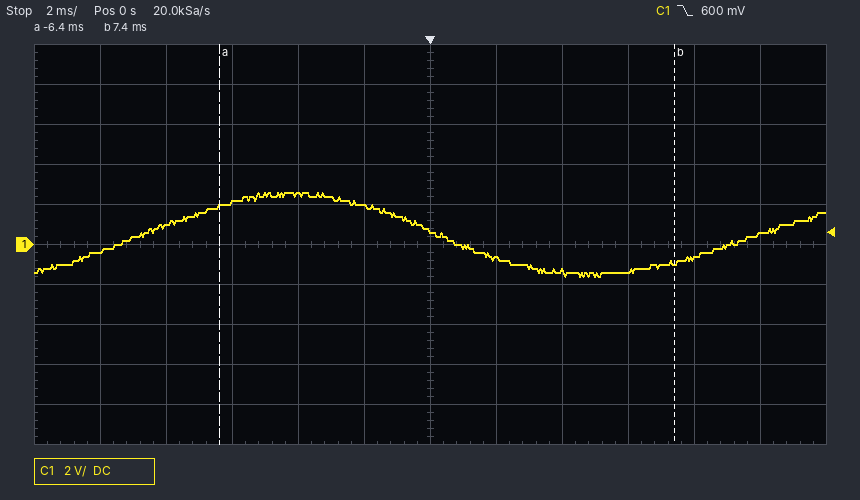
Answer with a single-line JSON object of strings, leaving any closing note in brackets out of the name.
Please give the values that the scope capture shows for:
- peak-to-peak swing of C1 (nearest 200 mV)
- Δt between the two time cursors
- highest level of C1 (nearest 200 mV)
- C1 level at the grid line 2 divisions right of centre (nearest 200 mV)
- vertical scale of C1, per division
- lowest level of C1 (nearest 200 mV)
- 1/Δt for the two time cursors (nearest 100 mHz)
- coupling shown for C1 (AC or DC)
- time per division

{"peak-to-peak swing of C1": "4.2 V", "Δt between the two time cursors": "13.8 ms", "highest level of C1": "2.6 V", "C1 level at the grid line 2 divisions right of centre": "-1.4 V", "vertical scale of C1, per division": "2 V", "lowest level of C1": "-1.6 V", "1/Δt for the two time cursors": "72.5 Hz", "coupling shown for C1": "DC", "time per division": "2 ms"}
